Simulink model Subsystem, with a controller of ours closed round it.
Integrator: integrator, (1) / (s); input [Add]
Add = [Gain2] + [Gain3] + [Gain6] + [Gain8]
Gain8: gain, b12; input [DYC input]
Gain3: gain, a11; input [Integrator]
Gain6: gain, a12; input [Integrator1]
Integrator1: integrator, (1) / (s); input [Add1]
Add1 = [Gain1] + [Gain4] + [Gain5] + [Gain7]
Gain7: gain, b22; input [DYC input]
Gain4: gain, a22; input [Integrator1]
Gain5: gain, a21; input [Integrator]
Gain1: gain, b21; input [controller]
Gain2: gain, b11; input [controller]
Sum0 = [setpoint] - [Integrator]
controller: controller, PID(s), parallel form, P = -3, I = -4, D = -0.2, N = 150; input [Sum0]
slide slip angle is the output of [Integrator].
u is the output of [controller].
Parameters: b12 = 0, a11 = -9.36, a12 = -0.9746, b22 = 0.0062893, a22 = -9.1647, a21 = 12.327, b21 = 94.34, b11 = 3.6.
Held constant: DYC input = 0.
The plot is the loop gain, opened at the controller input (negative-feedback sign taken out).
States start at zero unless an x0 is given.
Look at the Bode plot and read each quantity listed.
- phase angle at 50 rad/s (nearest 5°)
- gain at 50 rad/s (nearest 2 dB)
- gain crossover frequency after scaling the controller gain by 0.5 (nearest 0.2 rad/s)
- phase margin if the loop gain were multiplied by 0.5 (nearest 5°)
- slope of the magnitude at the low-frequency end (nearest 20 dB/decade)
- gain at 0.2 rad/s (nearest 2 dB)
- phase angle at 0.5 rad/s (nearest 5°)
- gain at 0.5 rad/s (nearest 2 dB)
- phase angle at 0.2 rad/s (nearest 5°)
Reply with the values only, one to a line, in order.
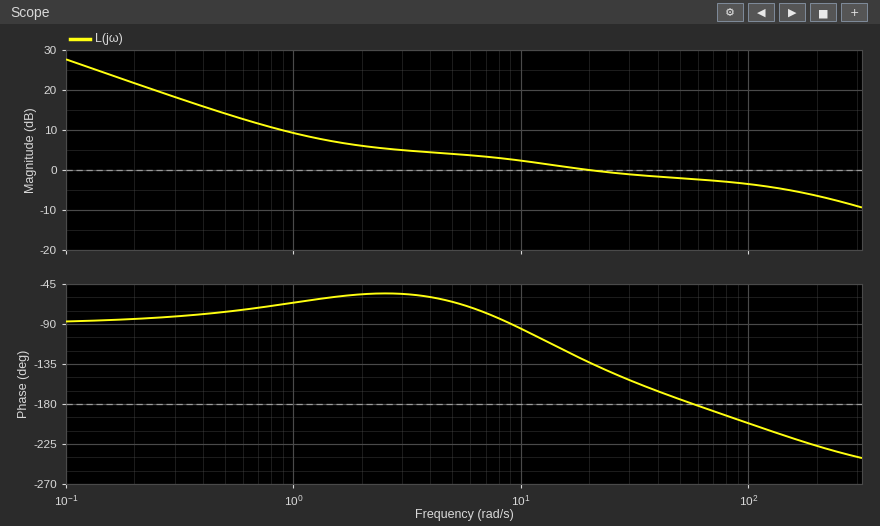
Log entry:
-175°
-2 dB
2.0 rad/s
125°
-20 dB/decade
22 dB
-75°
14 dB
-85°
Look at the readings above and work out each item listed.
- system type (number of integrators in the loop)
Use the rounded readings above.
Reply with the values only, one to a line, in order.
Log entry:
1
